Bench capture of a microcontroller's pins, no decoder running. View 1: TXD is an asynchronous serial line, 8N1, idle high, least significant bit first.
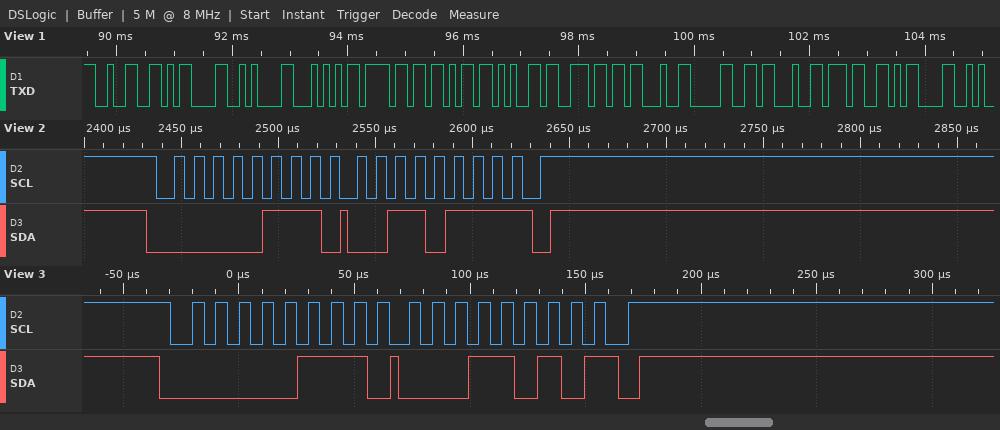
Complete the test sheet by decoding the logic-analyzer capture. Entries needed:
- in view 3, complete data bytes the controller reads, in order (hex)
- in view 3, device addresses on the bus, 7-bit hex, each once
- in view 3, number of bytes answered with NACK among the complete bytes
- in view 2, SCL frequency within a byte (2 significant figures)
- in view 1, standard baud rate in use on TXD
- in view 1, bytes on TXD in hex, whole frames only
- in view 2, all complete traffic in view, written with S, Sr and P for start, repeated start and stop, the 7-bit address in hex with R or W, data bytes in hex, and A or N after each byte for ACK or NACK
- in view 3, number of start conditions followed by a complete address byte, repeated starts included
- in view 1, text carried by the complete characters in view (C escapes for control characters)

1A
0x03
1
100 kHz
9600 baud
0x32 0x0D 0x0A 0x54 0x6F 0x6B 0x65 0x6E 0x23 0x30 0x23 0x37 0x0D
S 03R A 37 N P
1
"2\r\nToken#0#7\r"
